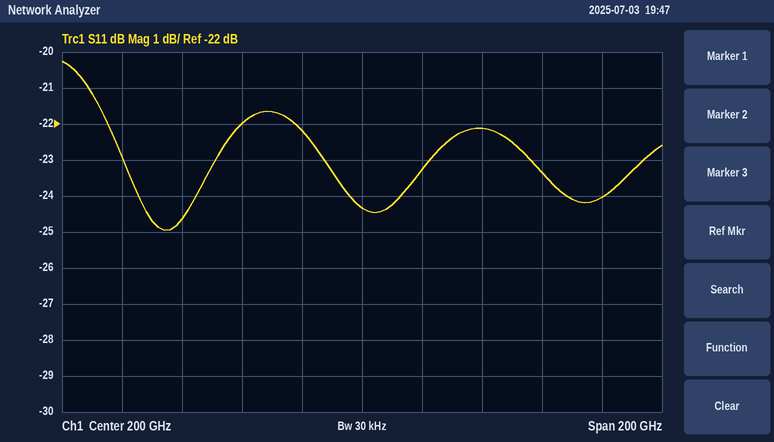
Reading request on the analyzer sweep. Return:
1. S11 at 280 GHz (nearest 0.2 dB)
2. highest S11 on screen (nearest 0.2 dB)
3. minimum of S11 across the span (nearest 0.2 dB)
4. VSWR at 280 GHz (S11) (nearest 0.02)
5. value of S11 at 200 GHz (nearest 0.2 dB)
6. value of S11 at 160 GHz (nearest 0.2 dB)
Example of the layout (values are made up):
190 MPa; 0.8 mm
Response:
-24.0 dB; -20.2 dB; -25.0 dB; 1.14; -24.4 dB; -22.0 dB
